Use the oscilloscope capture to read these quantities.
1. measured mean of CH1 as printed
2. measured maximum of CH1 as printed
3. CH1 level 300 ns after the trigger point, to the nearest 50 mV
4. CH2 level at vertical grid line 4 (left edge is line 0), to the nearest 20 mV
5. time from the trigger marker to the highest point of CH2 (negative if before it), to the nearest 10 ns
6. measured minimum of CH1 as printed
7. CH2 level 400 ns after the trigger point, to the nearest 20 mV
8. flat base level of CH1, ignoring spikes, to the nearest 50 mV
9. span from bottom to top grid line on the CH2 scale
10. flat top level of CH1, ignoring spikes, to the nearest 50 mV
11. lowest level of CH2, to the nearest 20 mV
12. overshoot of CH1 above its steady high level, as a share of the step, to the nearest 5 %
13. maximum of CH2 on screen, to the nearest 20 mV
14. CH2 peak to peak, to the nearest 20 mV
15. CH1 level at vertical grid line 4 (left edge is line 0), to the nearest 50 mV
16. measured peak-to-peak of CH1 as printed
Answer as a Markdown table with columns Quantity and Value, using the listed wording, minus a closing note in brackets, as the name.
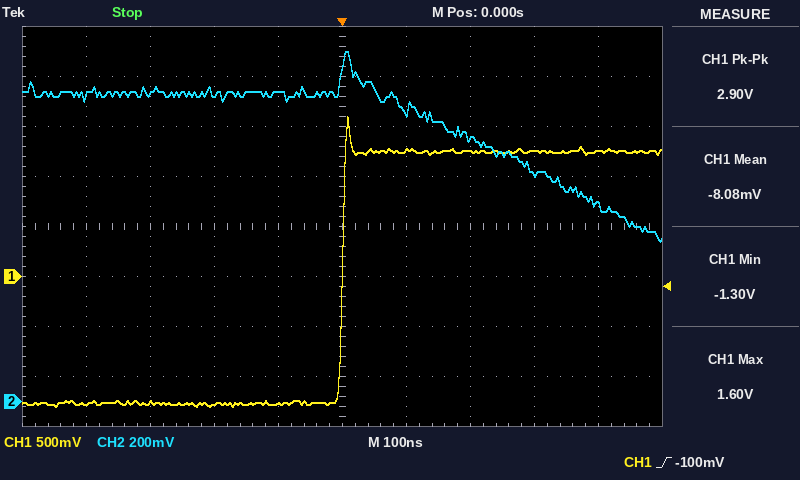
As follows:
| Quantity | Value |
|---|---|
| measured mean of CH1 as printed | -8.08 mV |
| measured maximum of CH1 as printed | 1.60 V |
| CH1 level 300 ns after the trigger point, to the nearest 50 mV | 1.25 V |
| CH2 level at vertical grid line 4 (left edge is line 0), to the nearest 20 mV | 1.24 V |
| time from the trigger marker to the highest point of CH2 (negative if before it), to the nearest 10 ns | +10 ns |
| measured minimum of CH1 as printed | -1.30 V |
| CH2 level 400 ns after the trigger point, to the nearest 20 mV | 780 mV |
| flat base level of CH1, ignoring spikes, to the nearest 50 mV | -1.25 V |
| span from bottom to top grid line on the CH2 scale | 1.6 V |
| flat top level of CH1, ignoring spikes, to the nearest 50 mV | 1.25 V |
| lowest level of CH2, to the nearest 20 mV | 640 mV |
| overshoot of CH1 above its steady high level, as a share of the step, to the nearest 5 % | 15 % |
| maximum of CH2 on screen, to the nearest 20 mV | 1.40 V |
| CH2 peak to peak, to the nearest 20 mV | 760 mV |
| CH1 level at vertical grid line 4 (left edge is line 0), to the nearest 50 mV | -1.25 V |
| measured peak-to-peak of CH1 as printed | 2.90 V |
